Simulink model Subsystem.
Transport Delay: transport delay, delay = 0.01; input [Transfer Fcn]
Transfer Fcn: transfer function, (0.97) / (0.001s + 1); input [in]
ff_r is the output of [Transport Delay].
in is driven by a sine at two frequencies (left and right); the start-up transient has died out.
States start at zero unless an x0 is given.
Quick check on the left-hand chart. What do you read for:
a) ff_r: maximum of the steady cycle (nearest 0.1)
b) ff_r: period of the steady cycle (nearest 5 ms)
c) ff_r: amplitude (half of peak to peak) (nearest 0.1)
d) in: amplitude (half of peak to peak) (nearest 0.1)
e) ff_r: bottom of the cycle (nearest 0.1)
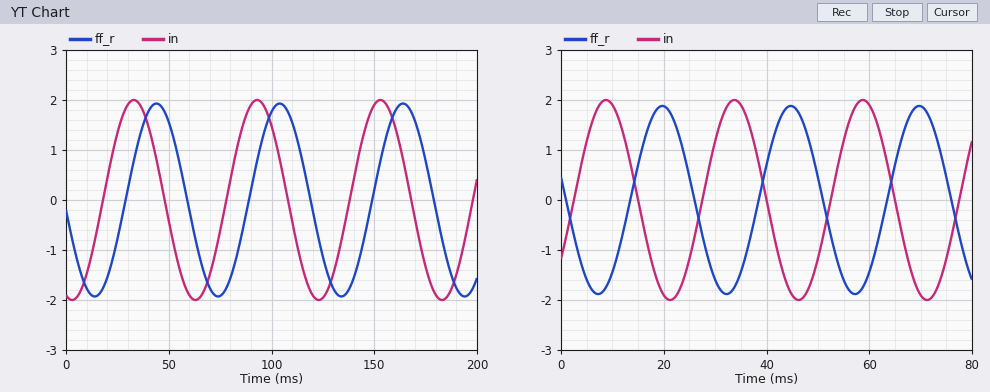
1.9
60 ms
1.9
2.0
-1.9
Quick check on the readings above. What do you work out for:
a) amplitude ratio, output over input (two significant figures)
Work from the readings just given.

0.95
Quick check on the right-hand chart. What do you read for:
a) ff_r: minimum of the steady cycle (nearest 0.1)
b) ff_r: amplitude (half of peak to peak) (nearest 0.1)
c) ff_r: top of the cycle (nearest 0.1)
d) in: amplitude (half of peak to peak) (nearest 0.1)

-1.9
1.9
1.9
2.0
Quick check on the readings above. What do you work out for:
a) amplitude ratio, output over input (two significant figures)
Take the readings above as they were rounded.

0.95
